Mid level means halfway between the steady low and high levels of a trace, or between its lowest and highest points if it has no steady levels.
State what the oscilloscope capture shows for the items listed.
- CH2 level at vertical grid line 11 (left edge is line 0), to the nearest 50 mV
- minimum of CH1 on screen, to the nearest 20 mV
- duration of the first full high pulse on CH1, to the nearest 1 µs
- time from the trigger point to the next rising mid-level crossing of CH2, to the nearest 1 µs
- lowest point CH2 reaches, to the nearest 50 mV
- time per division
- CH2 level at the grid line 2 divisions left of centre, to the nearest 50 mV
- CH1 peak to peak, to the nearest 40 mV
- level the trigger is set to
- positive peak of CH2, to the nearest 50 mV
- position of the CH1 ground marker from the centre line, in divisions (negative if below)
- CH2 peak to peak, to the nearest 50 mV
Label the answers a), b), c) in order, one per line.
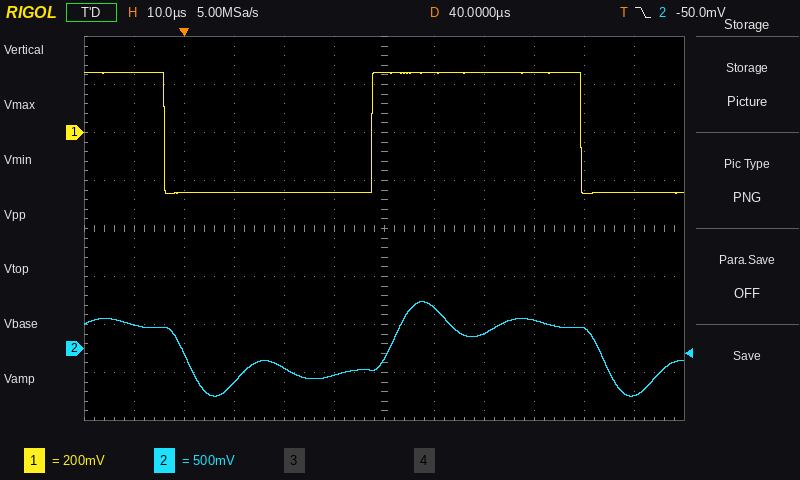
a) -500 mV
b) -260 mV
c) 42 µs
d) 41 µs
e) -500 mV
f) 10 µs
g) -200 mV
h) 520 mV
i) -50.0 mV
j) 500 mV
k) +2.0 div
l) 1.00 V
